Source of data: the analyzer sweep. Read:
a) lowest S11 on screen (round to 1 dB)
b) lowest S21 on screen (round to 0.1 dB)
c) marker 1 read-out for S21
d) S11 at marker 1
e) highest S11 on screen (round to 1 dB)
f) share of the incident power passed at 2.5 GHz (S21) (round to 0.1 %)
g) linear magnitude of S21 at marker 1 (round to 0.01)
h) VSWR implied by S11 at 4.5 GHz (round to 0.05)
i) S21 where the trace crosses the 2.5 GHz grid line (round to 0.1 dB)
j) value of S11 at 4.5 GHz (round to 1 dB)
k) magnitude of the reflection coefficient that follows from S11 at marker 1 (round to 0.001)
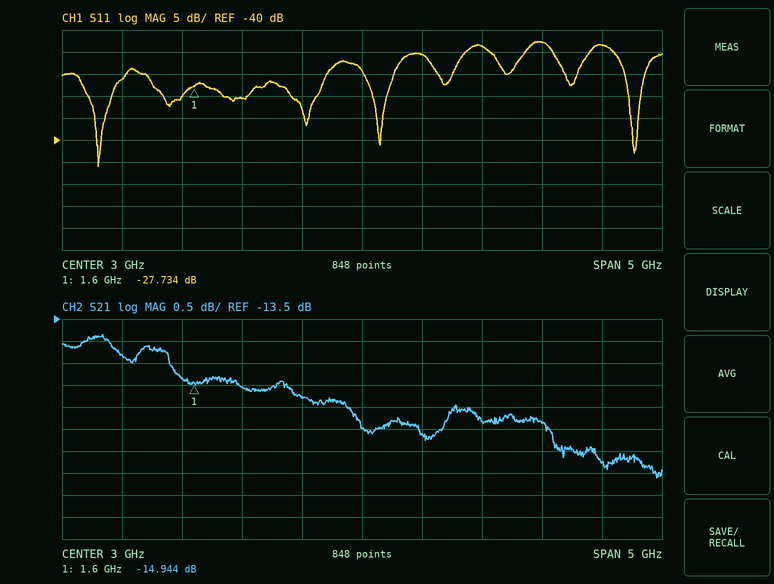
-46 dB
-17.1 dB
-14.944 dB
-27.734 dB
-18 dB
3.0 %
0.18
1.30
-15.3 dB
-18 dB
0.041
